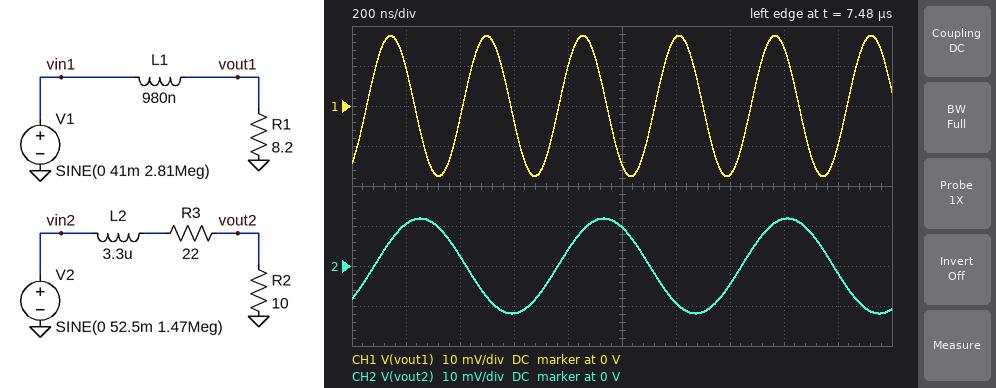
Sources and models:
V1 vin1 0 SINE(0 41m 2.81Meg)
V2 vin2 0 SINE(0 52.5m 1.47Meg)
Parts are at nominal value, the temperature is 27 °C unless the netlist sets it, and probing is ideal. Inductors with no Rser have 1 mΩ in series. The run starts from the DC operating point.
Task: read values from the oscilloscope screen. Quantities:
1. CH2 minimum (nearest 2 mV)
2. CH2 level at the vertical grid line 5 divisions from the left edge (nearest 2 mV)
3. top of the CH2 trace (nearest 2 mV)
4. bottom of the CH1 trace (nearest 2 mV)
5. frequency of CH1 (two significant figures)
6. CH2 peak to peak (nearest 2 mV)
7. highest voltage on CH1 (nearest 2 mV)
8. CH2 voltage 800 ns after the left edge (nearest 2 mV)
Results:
-12 mV
10 mV
12 mV
-18 mV
2.8 MHz
24 mV
18 mV
4 mV
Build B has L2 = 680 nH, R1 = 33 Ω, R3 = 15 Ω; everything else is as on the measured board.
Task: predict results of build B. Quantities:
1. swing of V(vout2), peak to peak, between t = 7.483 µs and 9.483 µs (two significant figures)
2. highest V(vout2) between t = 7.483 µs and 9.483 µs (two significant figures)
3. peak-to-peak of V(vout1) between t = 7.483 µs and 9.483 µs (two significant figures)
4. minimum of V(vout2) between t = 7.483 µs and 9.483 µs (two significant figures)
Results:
41 mV
20 mV
73 mV
-20 mV
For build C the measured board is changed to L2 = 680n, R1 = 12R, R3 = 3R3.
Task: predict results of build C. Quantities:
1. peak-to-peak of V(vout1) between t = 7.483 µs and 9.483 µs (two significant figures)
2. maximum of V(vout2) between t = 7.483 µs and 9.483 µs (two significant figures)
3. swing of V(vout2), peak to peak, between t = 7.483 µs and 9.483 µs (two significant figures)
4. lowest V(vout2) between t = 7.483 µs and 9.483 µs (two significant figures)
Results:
47 mV
36 mV
71 mV
-36 mV
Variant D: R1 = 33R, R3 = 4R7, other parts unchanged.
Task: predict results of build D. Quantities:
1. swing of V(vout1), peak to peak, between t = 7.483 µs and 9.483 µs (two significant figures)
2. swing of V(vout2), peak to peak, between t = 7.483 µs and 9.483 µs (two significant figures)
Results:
73 mV
31 mV
